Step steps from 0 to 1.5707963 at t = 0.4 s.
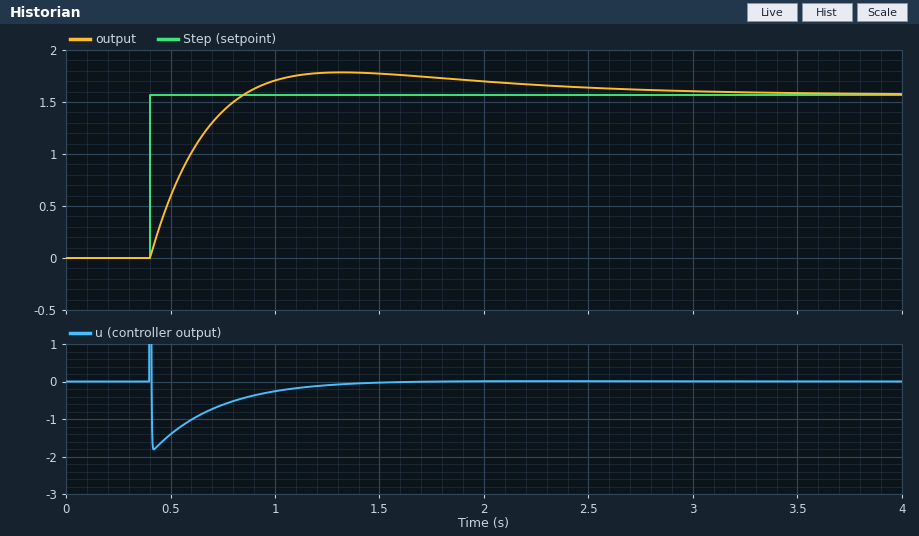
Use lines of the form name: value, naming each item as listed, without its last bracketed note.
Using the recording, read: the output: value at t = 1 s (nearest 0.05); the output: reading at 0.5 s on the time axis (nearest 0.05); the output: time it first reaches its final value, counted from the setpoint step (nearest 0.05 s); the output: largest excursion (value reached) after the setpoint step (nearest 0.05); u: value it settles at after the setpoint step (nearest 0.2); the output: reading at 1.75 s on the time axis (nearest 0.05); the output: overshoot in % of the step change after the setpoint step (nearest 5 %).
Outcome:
the output: value at t = 1 s: 1.70
the output: reading at 0.5 s on the time axis: 0.60
the output: time it first reaches its final value, counted from the setpoint step: 0.45 s
the output: largest excursion (value reached) after the setpoint step: 1.80
u: value it settles at after the setpoint step: 0.0
the output: reading at 1.75 s on the time axis: 1.75
the output: overshoot in % of the step change after the setpoint step: 15 %
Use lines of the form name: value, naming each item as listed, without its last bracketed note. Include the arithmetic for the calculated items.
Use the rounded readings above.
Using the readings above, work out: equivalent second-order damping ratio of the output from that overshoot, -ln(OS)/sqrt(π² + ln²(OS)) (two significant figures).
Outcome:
equivalent second-order damping ratio of the output from that overshoot, -ln(OS)/sqrt(π² + ln²(OS)): ln(0.15) = -1.897; 1.897 / sqrt(9.870 + 3.599) = 0.52
